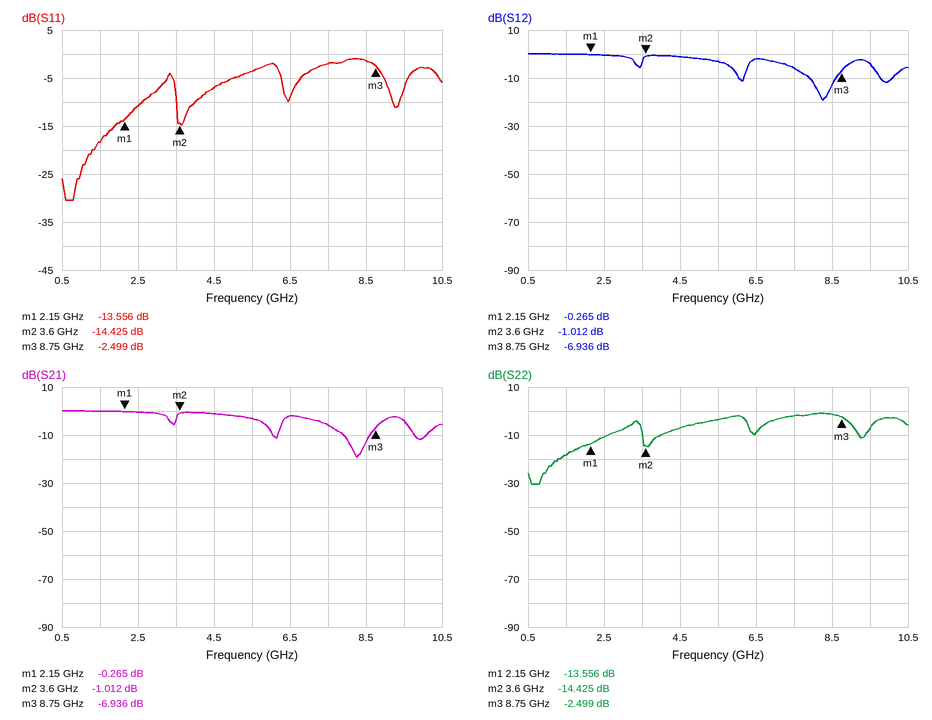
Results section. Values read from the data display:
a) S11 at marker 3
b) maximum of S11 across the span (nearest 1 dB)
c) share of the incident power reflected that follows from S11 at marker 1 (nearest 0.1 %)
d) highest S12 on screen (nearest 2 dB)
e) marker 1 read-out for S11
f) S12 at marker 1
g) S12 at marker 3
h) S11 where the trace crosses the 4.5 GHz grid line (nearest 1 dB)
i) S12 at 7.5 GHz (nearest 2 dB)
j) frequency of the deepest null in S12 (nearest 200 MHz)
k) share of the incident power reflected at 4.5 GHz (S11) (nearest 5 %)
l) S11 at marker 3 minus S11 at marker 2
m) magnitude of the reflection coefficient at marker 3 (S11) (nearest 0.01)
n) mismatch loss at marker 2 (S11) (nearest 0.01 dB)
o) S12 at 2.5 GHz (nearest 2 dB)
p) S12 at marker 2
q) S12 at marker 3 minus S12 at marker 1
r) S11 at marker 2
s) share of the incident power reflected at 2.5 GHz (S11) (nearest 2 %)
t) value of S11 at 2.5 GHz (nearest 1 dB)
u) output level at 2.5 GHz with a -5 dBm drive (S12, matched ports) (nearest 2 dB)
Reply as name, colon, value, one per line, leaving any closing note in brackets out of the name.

S11 at marker 3: -2.499 dB
maximum of S11 across the span: -1 dB
share of the incident power reflected that follows from S11 at marker 1: 4.4 %
highest S12 on screen: 0 dB
marker 1 read-out for S11: -13.556 dB
S12 at marker 1: -0.265 dB
S12 at marker 3: -6.936 dB
S11 where the trace crosses the 4.5 GHz grid line: -7 dB
S12 at 7.5 GHz: -6 dB
frequency of the deepest null in S12: 8.2 GHz
share of the incident power reflected at 4.5 GHz (S11): 20 %
S11 at marker 3 minus S11 at marker 2: 11.926 dB
magnitude of the reflection coefficient at marker 3 (S11): 0.75
mismatch loss at marker 2 (S11): 0.16 dB
S12 at 2.5 GHz: 0 dB
S12 at marker 2: -1.012 dB
S12 at marker 3 minus S12 at marker 1: -6.671 dB
S11 at marker 2: -14.425 dB
share of the incident power reflected at 2.5 GHz (S11): 8 %
value of S11 at 2.5 GHz: -11 dB
output level at 2.5 GHz with a -5 dBm drive (S12, matched ports): -6 dBm
